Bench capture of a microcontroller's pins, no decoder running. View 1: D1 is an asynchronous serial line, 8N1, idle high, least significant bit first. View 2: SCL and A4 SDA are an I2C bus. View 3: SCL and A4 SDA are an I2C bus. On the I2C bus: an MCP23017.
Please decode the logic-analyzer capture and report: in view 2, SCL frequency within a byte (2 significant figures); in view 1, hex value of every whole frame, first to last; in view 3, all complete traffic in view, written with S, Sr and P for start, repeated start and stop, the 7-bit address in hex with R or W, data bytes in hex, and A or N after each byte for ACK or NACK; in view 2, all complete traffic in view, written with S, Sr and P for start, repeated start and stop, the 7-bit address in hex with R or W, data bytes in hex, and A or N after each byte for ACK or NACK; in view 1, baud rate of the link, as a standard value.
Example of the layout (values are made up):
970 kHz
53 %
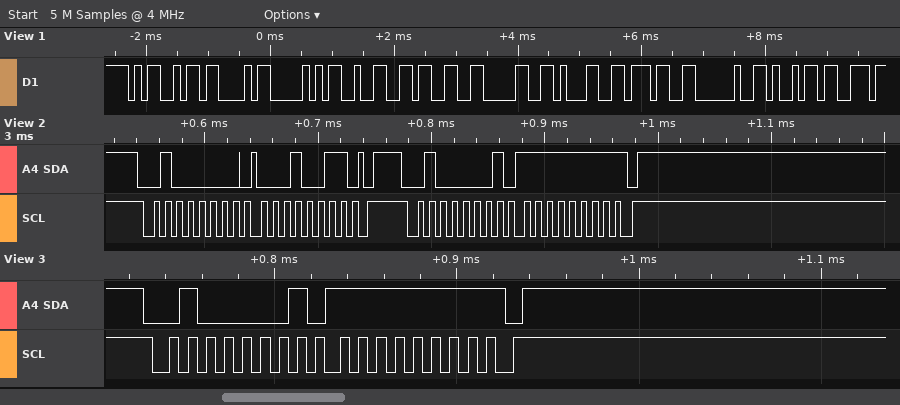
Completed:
100 kHz
0x4D 0x43 0x50 0x32 0x33 0x30 0x31 0x37 0x20 0x69
S 20R A FF N P
S 20W A 13 A P S 20R A FF N P
9600 baud
